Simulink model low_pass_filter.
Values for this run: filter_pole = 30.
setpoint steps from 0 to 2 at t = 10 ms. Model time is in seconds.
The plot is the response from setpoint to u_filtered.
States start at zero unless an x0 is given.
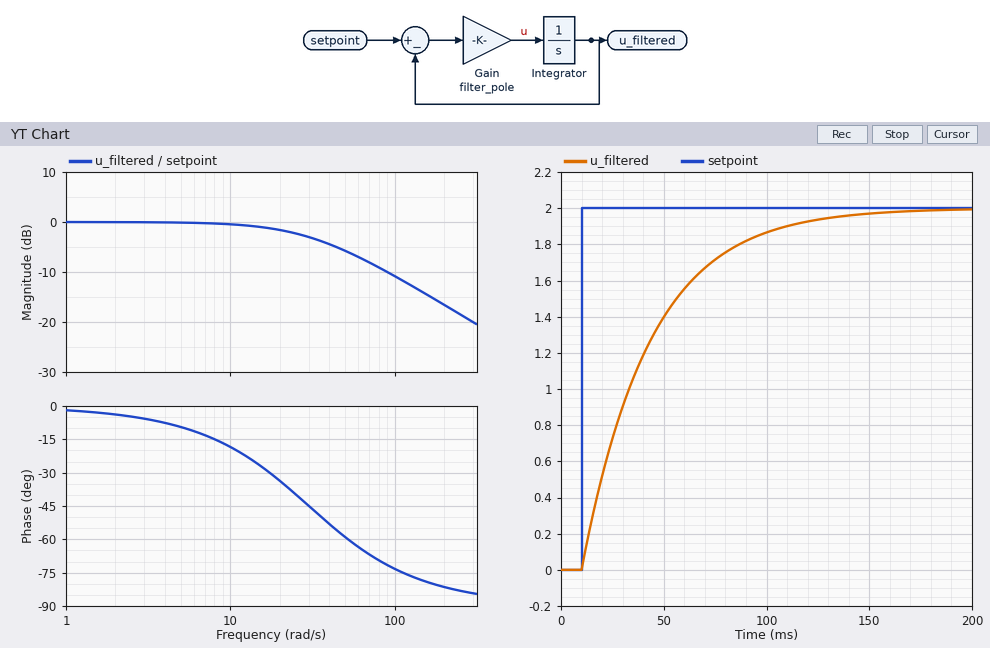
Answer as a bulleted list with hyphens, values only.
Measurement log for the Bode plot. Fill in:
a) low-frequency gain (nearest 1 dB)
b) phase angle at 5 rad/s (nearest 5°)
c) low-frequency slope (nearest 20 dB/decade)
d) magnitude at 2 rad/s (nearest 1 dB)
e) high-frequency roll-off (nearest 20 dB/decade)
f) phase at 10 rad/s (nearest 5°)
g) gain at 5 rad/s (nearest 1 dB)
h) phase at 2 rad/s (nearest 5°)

- 0 dB
- -10°
- 0 dB/decade
- 0 dB
- -20 dB/decade
- -20°
- 0 dB
- -5°
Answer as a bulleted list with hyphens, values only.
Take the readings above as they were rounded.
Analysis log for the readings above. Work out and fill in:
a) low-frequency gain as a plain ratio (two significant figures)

- 1.0
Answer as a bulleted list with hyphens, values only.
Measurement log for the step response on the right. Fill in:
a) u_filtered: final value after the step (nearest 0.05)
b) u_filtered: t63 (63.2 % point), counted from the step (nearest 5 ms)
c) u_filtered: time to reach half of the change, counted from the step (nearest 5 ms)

- 2.00
- 35 ms
- 25 ms
